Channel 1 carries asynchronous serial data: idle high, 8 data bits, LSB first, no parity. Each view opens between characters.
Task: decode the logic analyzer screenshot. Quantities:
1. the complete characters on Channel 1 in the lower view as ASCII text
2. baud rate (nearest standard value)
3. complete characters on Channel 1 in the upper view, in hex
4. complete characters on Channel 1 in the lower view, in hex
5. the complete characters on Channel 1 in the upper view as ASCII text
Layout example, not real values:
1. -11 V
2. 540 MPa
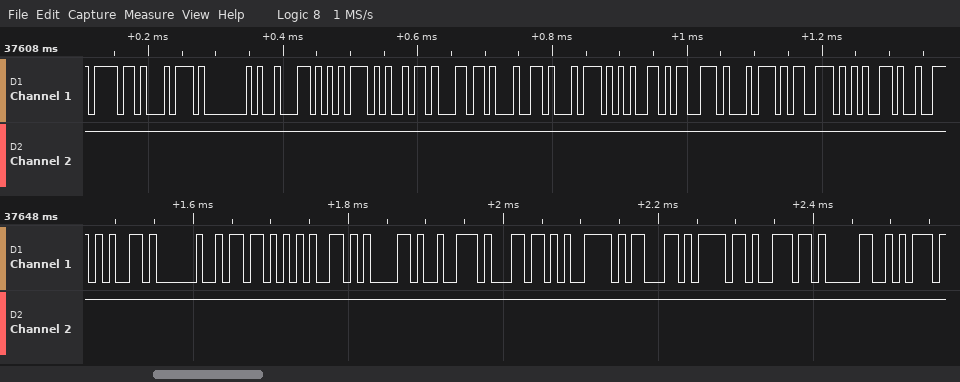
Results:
1. "e [earlycon0"
2. 115200 baud
3. 6F, 74, 40, 62, 75, 69, 6C, 64, 74, 65, 73, 74, 73, 65
4. 65, 20, 5B, 65, 61, 72, 6C, 79, 63, 6F, 6E, 30
5. "ot@buildtestse"
